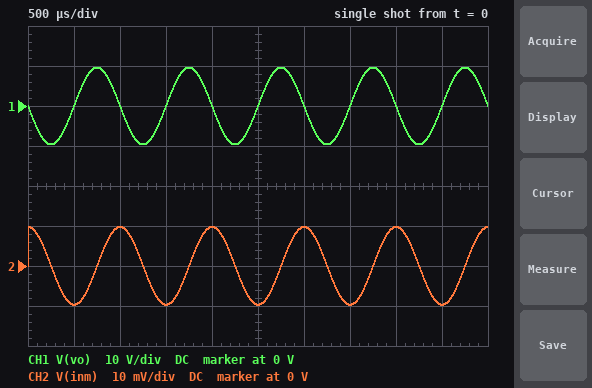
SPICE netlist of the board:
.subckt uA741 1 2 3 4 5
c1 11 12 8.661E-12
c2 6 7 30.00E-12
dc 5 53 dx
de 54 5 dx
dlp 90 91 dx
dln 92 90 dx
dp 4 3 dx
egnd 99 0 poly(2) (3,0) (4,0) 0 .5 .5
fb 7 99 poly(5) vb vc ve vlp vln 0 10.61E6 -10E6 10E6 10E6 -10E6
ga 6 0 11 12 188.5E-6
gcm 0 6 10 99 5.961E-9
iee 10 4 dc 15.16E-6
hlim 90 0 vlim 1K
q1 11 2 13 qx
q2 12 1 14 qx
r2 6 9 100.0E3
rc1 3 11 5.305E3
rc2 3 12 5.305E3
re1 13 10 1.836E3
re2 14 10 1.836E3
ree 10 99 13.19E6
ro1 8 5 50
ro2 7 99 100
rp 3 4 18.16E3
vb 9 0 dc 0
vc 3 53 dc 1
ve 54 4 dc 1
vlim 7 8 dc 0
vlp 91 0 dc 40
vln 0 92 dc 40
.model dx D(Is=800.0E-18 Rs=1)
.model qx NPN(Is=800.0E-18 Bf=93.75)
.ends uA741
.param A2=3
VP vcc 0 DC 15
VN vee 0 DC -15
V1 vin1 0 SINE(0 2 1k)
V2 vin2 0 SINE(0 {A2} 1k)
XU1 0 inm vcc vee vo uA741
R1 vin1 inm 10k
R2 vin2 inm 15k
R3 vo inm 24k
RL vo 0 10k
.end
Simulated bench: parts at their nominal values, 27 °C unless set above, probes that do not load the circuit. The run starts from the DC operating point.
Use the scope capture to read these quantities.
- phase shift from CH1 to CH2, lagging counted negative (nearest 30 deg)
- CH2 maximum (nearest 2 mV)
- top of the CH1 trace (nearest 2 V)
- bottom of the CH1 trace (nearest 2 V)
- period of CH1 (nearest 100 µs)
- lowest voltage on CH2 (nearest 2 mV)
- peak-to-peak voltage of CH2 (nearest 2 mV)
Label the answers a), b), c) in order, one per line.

a) -90 deg
b) 10 mV
c) 10 V
d) -10 V
e) 1.0 ms
f) -10 mV
g) 20 mV
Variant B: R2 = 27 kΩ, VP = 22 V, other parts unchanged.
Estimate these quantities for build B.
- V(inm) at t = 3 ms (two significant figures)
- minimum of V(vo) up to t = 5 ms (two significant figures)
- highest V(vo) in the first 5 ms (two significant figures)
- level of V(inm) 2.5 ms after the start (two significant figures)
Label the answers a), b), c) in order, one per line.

a) 7.8 mV
b) -7.5 V
c) 7.5 V
d) -7.5 mV
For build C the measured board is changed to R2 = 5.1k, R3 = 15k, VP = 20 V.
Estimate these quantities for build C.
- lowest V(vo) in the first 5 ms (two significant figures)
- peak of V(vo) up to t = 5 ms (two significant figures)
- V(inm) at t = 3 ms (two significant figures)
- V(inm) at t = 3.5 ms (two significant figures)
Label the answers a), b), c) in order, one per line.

a) -12 V
b) 12 V
c) 12 mV
d) -12 mV
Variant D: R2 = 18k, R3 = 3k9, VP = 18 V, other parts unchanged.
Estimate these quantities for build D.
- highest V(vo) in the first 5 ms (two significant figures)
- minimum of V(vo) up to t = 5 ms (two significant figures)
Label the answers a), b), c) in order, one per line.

a) 1.4 V
b) -1.4 V
